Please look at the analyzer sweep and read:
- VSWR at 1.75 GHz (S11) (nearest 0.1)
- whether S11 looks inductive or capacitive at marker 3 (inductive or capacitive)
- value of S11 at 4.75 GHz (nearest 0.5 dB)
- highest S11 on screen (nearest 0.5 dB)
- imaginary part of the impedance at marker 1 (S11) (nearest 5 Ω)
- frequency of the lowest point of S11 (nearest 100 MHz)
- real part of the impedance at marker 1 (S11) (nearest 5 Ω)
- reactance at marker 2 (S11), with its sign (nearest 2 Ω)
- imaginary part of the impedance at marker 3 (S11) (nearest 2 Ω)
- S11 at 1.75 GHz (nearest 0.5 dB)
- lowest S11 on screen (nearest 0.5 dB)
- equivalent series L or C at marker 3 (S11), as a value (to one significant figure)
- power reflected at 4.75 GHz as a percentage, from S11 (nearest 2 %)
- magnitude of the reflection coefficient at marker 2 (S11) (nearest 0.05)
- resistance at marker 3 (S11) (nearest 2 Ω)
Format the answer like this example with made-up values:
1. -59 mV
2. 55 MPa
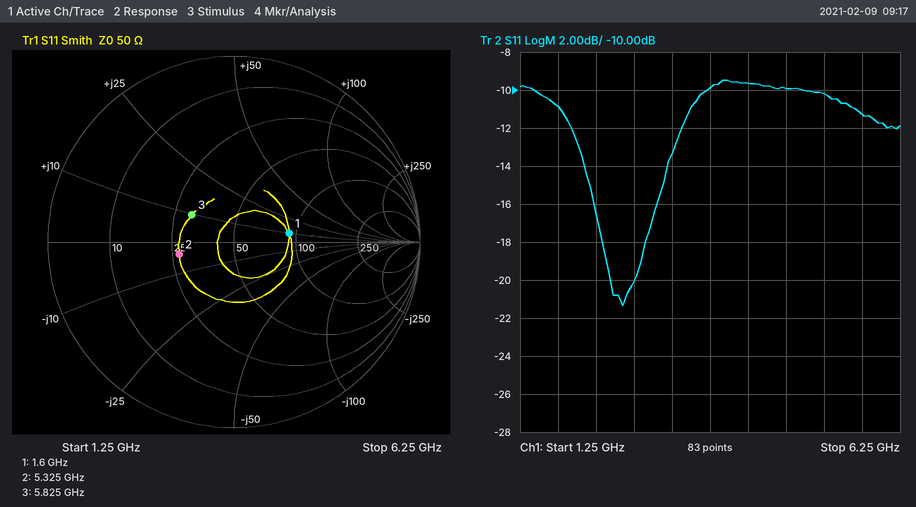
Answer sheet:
1. 1.8
2. inductive
3. -10.0 dB
4. -9.5 dB
5. +10 Ω
6. 2.6 GHz
7. 90 Ω
8. -4 Ω
9. +10 Ω
10. -11.0 dB
11. -21.5 dB
12. 300 pH
13. 10 %
14. 0.30
15. 30 Ω
